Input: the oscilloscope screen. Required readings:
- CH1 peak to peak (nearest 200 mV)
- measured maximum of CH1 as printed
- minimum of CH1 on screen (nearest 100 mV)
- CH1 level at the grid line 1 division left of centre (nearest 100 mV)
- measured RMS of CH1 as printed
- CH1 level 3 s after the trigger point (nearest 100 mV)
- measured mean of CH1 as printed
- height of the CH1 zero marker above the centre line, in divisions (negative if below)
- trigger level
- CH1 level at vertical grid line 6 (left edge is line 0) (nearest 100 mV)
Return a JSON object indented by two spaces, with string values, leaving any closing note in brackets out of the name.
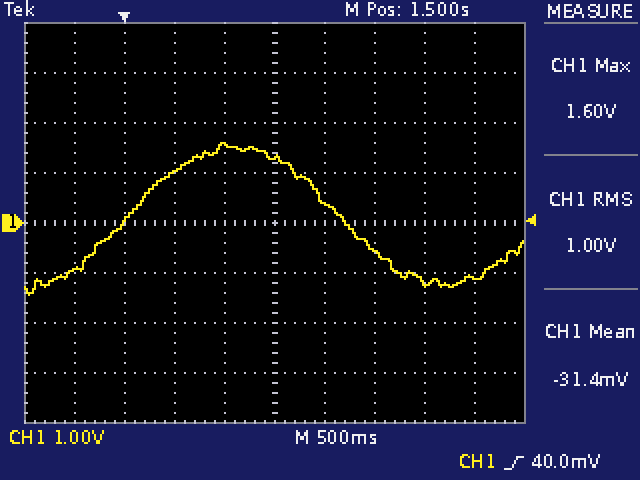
{
  "CH1 peak to peak": "3.0 V",
  "measured maximum of CH1 as printed": "1.60 V",
  "minimum of CH1 on screen": "-1.4 V",
  "CH1 level at the grid line 1 division left of centre": "1.6 V",
  "measured RMS of CH1 as printed": "1.00 V",
  "CH1 level 3 s after the trigger point": "-1.2 V",
  "measured mean of CH1 as printed": "-31.4 mV",
  "height of the CH1 zero marker above the centre line, in divisions": "0.0 div",
  "trigger level": "40.0 mV",
  "CH1 level at vertical grid line 6 (left edge is line 0)": "400 mV"
}
